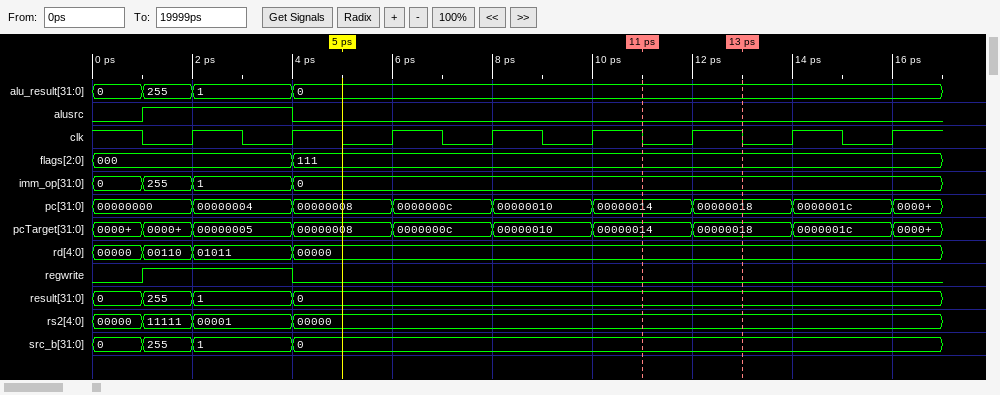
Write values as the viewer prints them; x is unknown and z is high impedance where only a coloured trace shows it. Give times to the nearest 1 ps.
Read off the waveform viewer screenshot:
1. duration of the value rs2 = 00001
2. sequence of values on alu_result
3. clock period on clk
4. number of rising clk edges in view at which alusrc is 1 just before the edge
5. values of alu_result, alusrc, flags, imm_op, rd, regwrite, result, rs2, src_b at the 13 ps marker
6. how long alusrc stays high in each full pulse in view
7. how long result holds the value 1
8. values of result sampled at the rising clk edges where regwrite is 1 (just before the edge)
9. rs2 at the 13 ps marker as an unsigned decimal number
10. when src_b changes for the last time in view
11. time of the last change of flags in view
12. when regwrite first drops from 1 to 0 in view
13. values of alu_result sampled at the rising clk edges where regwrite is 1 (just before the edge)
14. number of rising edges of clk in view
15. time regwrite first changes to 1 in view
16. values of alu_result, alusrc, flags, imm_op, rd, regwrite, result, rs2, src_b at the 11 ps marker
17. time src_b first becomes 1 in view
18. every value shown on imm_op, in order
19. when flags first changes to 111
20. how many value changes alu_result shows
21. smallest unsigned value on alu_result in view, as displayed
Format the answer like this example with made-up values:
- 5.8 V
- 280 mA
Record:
- 2 ps
- 0, 255, 1, 0
- 2 ps
- 2
- alu_result=0, alusrc=0, flags=111, imm_op=0, rd=00000, regwrite=0, result=0, rs2=00000, src_b=0
- 3 ps
- 2 ps
- 255, 1
- 0
- 4 ps
- 4 ps
- 4 ps
- 255, 1
- 8
- 1 ps
- alu_result=0, alusrc=0, flags=111, imm_op=0, rd=00000, regwrite=0, result=0, rs2=00000, src_b=0
- 2 ps
- 0, 255, 1, 0
- 4 ps
- 3
- 0
